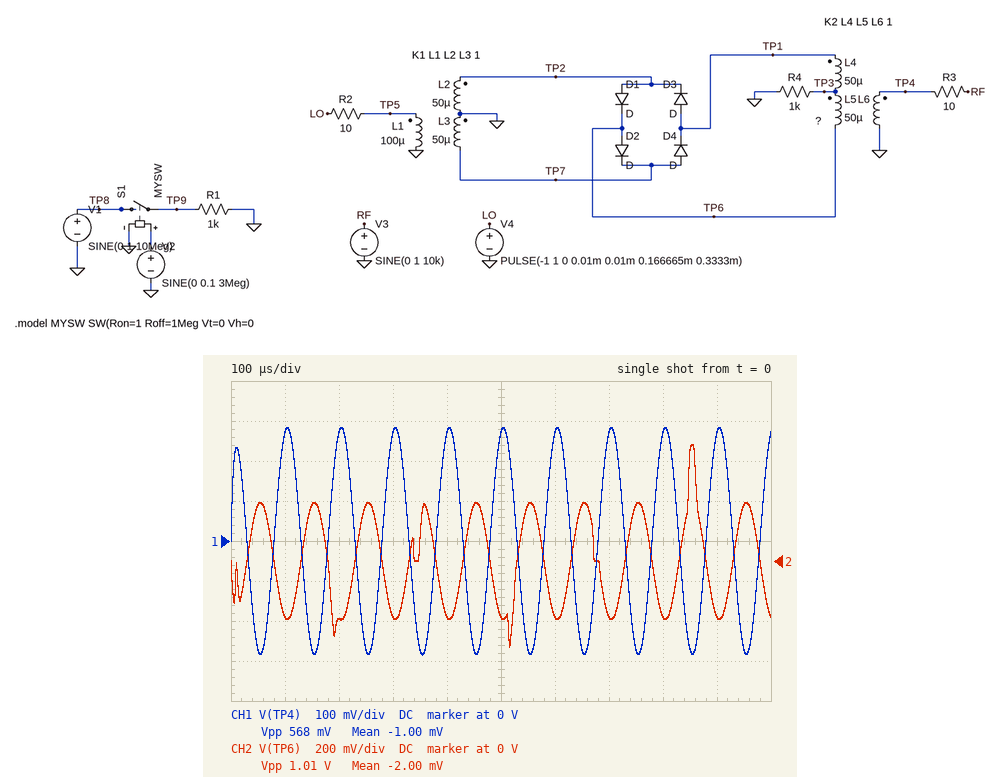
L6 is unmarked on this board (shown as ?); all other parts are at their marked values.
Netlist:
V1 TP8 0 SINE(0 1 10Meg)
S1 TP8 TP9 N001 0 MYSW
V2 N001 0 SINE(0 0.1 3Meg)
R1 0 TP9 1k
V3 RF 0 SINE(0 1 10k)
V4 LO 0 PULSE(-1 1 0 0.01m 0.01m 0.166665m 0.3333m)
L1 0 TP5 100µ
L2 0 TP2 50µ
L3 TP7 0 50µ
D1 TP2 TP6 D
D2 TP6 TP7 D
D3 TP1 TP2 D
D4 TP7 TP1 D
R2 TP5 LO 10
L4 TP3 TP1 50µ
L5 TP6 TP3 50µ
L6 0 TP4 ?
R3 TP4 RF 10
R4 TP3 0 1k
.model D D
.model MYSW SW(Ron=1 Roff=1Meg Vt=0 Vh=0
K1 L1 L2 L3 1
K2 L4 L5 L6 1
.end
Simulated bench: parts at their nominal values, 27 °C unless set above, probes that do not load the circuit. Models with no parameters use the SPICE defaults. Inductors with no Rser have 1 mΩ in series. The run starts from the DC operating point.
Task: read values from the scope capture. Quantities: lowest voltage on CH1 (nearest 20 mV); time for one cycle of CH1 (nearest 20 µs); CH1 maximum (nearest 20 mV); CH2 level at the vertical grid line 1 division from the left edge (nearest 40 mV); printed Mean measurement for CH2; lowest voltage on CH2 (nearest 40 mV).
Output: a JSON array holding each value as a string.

["-280 mV", "100 µs", "280 mV", "-280 mV", "-2.00 mV", "-440 mV"]
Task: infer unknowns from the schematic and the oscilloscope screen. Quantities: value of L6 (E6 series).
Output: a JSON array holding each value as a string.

["47 µH"]
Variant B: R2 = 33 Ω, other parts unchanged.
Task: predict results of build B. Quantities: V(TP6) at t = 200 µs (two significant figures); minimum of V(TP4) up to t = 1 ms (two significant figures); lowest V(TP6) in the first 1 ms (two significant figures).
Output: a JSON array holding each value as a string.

["-280 mV", "-280 mV", "-290 mV"]
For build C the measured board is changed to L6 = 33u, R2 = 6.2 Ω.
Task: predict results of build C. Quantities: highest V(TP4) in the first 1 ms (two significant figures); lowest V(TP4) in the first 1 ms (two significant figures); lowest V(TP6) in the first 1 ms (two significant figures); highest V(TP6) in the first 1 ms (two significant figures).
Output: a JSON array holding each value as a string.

["200 mV", "-200 mV", "-450 mV", "500 mV"]
